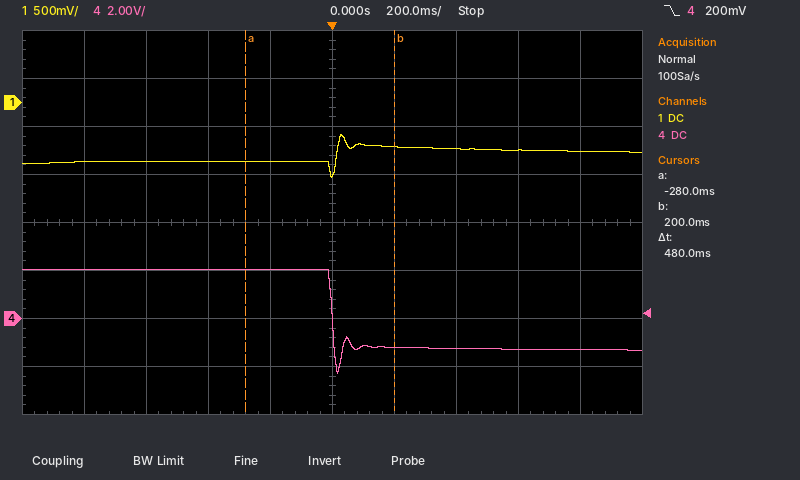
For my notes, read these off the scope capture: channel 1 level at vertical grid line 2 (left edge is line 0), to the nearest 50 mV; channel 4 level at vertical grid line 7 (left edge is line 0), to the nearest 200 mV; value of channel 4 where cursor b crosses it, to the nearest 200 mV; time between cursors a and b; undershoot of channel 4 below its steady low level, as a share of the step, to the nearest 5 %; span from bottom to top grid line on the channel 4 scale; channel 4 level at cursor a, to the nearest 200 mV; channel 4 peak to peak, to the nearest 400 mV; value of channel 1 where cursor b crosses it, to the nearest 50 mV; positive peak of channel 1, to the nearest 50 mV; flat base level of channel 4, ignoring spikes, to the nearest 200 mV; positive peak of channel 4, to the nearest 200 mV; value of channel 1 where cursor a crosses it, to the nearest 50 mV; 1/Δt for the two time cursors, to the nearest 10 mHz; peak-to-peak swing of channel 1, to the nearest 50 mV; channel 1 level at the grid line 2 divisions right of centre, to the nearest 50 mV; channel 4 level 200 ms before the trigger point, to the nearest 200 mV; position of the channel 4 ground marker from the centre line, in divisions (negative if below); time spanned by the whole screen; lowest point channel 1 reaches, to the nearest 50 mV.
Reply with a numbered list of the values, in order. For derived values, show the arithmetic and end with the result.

1. -600 mV
2. -1.2 V
3. -1.2 V
4. 480 ms
5. 30 %
6. 16 V
7. 2.0 V
8. 4.4 V
9. -450 mV
10. -350 mV
11. -1.2 V
12. 2.0 V
13. -600 mV
14. 1 / 480 ms ≈ 2.08 Hz
15. -350 mV − (-800 mV) = 450 mV
16. -500 mV
17. 2.0 V
18. -2.0 div
19. 2 s
20. -800 mV
